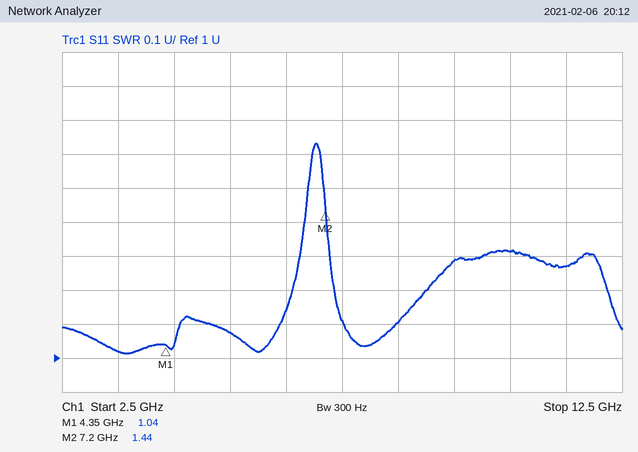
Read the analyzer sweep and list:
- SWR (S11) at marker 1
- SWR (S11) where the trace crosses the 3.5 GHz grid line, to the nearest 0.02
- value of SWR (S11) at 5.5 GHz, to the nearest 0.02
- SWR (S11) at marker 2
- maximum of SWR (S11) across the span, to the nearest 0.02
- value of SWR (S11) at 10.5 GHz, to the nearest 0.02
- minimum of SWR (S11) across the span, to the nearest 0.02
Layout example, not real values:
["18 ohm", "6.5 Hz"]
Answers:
["1.04", "1.02", "1.08", "1.44", "1.64", "1.32", "1.02"]
